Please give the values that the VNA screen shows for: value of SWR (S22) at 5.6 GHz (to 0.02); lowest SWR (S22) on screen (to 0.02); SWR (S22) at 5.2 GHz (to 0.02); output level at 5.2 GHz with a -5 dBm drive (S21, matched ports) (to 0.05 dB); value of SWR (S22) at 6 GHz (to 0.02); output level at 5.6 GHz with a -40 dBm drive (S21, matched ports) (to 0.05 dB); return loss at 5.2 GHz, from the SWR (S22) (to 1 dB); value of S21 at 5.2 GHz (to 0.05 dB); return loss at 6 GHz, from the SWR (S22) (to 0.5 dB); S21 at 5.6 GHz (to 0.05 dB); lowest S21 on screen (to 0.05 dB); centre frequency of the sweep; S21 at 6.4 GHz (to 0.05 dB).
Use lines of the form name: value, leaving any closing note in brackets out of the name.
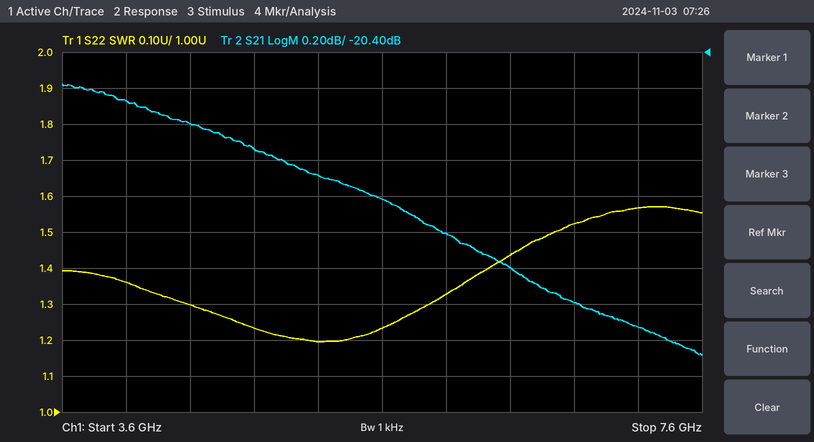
value of SWR (S22) at 5.6 GHz: 1.24
lowest SWR (S22) on screen: 1.20
SWR (S22) at 5.2 GHz: 1.20
output level at 5.2 GHz with a -5 dBm drive (S21, matched ports): -26.10 dBm
value of SWR (S22) at 6 GHz: 1.32
output level at 5.6 GHz with a -40 dBm drive (S21, matched ports): -61.20 dBm
return loss at 5.2 GHz, from the SWR (S22): 21 dB
value of S21 at 5.2 GHz: -21.10 dB
return loss at 6 GHz, from the SWR (S22): 17.0 dB
S21 at 5.6 GHz: -21.20 dB
lowest S21 on screen: -22.10 dB
centre frequency of the sweep: 5.6 GHz
S21 at 6.4 GHz: -21.60 dB
